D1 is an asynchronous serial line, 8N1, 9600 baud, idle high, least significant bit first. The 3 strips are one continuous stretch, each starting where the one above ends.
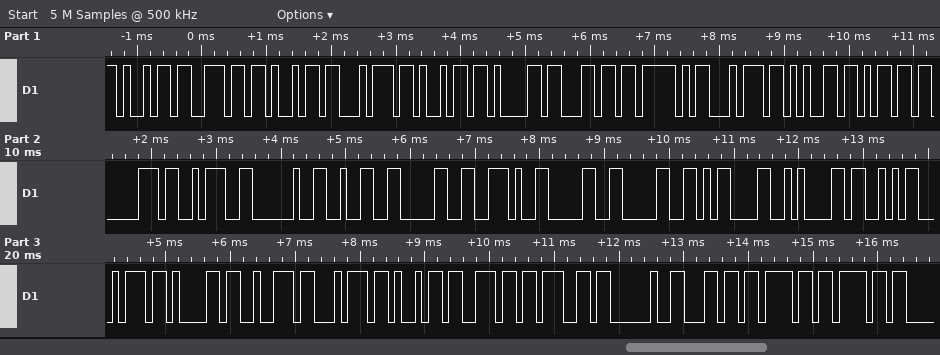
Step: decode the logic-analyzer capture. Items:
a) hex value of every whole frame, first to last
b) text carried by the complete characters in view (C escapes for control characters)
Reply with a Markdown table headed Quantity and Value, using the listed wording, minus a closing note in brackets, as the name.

| Quantity | Value |
|---|---|
| hex value of every whole frame, first to last | 69 6E 69 74 69 61 6C 5F 74 65 6D 70 3A 20 32 30 2E 30 30 0D 0A 53 74 61 72 74 69 6E 67 20 6C 6F 6F |
| text carried by the complete characters in view | "initial_temp: 20.00\r\nStarting loo" |
